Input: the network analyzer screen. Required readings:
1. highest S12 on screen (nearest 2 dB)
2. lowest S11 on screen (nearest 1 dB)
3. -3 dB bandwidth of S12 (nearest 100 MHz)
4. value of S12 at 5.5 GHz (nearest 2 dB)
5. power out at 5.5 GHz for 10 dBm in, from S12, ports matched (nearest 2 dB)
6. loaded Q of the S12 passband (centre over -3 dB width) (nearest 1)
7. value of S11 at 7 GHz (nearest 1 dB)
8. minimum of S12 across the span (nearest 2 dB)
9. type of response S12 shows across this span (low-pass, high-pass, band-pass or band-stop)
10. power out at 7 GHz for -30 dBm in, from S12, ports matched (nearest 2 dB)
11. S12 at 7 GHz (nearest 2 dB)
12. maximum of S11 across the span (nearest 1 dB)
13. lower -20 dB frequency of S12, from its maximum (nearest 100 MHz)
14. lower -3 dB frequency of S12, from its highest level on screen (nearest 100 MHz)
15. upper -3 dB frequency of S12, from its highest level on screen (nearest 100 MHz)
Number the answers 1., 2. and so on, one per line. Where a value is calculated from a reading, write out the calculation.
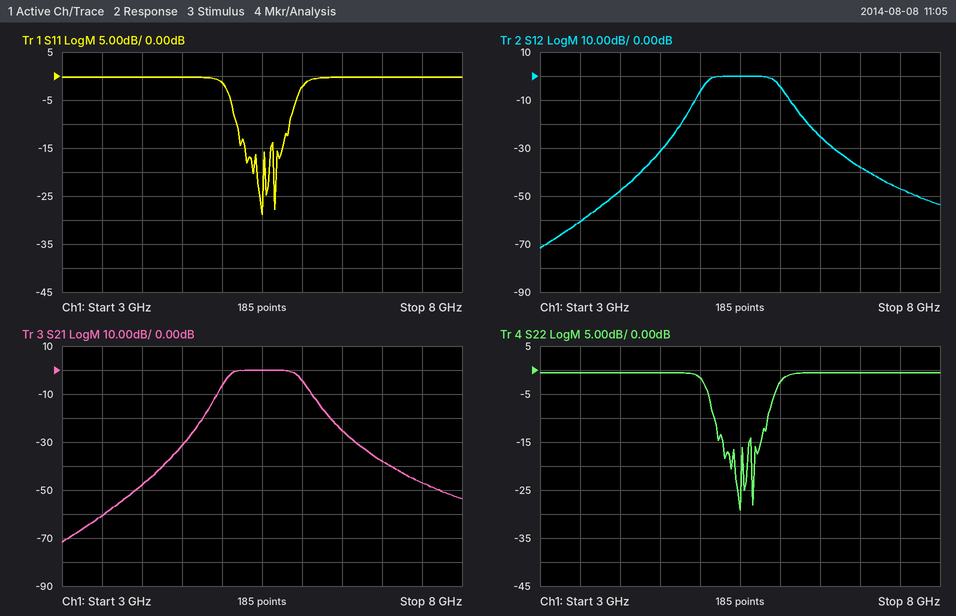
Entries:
1. 0 dB
2. -29 dB
3. 6.0 GHz − 5.1 GHz = 900 MHz
4. 0 dB
5. 10 dBm + (0 dB) = 10 dBm
6. 5.55 GHz / 900 MHz ≈ 6
7. 0 dB
8. -72 dB
9. band-pass
10. -30 dBm + (-38 dB) = -68 dBm
11. -38 dB
12. 0 dB
13. 4.8 GHz
14. 5.1 GHz
15. 6.0 GHz
